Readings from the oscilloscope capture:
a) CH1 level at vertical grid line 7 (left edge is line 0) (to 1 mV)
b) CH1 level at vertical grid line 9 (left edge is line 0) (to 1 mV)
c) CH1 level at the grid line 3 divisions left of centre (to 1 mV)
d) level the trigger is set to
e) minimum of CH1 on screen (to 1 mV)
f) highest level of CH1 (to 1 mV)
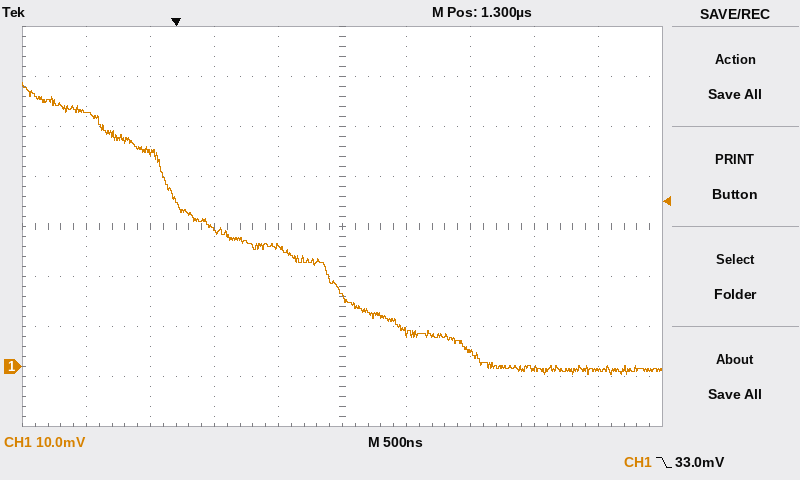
3 mV
-1 mV
43 mV
33.0 mV
-2 mV
57 mV
